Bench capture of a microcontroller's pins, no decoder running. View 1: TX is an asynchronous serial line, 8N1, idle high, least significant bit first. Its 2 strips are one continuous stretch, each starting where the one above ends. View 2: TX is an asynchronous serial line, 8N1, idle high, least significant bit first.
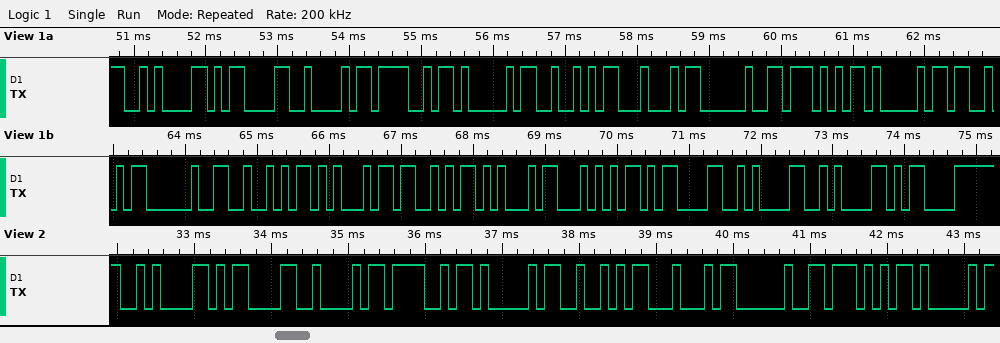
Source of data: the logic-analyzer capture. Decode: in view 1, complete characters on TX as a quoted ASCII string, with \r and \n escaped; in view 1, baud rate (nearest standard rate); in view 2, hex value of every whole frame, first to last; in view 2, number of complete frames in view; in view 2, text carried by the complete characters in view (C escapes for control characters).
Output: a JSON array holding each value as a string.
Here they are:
["\"\\n\\rBOARD WAS RESET\\r\\n\\n\\r\"", "9600 baud", "0A 0D 42 4F 41 52 44 20 57 41", "10", "\"\\n\\rBOARD WA\""]
